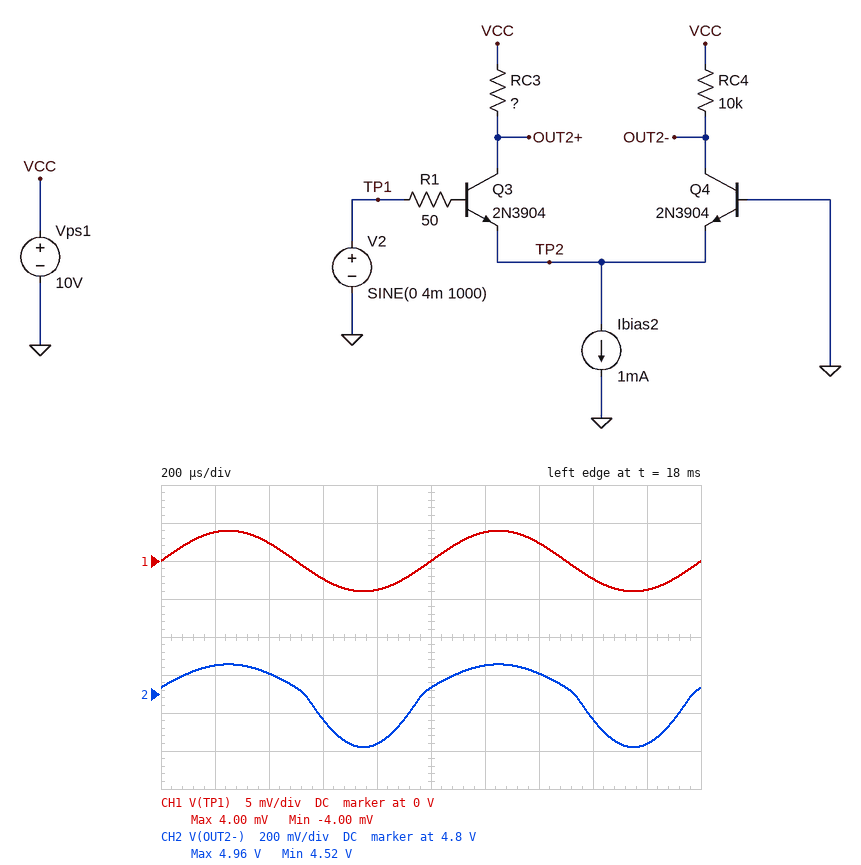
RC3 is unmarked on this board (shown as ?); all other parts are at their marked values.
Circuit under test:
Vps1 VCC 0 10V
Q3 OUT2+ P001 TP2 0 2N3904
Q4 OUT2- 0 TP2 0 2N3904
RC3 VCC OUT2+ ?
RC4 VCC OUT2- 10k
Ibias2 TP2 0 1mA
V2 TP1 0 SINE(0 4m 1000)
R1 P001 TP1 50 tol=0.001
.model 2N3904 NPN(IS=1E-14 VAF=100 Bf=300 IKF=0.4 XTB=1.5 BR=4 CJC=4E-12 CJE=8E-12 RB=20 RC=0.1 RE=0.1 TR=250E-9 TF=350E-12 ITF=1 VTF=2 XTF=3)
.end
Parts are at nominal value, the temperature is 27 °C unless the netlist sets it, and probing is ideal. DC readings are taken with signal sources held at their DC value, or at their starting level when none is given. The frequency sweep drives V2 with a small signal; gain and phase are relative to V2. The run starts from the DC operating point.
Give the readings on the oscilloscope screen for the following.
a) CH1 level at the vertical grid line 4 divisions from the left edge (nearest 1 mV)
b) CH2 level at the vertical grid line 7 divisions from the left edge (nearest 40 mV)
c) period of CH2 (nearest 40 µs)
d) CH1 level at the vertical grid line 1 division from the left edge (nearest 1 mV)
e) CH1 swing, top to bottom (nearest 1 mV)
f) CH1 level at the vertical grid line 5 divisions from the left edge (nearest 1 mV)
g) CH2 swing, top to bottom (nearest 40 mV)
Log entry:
-4 mV
4.92 V
1.00 ms
4 mV
8 mV
0 V
440 mV
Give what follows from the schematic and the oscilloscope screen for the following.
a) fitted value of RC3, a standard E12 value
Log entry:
22 kΩ
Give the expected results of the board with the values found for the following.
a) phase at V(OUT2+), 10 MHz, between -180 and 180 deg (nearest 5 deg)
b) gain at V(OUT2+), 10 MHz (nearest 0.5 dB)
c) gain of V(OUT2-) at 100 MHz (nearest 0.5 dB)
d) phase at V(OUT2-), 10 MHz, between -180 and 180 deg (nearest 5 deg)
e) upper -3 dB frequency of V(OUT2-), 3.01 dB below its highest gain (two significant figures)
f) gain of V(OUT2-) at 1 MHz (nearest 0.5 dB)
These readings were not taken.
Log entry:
60 deg
3.0 dB
11.5 dB
-55 deg
7.5 MHz
34.5 dB
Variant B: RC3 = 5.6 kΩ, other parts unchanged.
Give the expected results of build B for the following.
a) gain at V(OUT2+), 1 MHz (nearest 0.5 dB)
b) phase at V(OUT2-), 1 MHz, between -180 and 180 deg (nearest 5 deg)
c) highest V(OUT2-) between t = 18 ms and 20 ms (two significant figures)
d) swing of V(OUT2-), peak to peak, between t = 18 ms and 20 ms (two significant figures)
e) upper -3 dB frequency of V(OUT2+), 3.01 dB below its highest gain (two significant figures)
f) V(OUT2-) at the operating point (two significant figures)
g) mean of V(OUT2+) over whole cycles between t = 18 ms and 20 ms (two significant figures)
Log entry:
34.0 dB
-10 deg
5.4 V
740 mV
7.7 MHz
5.1 V
7.2 V
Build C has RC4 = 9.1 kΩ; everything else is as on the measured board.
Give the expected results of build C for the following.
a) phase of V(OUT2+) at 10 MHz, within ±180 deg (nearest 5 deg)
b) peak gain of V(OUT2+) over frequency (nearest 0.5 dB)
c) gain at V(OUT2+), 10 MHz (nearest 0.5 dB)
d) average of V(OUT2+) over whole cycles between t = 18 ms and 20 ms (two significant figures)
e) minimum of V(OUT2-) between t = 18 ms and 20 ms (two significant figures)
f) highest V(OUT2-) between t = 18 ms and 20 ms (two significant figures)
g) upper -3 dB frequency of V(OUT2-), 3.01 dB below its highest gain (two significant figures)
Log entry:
65 deg
31.5 dB
4.0 dB
-340 mV
5.0 V
5.4 V
8.4 MHz
